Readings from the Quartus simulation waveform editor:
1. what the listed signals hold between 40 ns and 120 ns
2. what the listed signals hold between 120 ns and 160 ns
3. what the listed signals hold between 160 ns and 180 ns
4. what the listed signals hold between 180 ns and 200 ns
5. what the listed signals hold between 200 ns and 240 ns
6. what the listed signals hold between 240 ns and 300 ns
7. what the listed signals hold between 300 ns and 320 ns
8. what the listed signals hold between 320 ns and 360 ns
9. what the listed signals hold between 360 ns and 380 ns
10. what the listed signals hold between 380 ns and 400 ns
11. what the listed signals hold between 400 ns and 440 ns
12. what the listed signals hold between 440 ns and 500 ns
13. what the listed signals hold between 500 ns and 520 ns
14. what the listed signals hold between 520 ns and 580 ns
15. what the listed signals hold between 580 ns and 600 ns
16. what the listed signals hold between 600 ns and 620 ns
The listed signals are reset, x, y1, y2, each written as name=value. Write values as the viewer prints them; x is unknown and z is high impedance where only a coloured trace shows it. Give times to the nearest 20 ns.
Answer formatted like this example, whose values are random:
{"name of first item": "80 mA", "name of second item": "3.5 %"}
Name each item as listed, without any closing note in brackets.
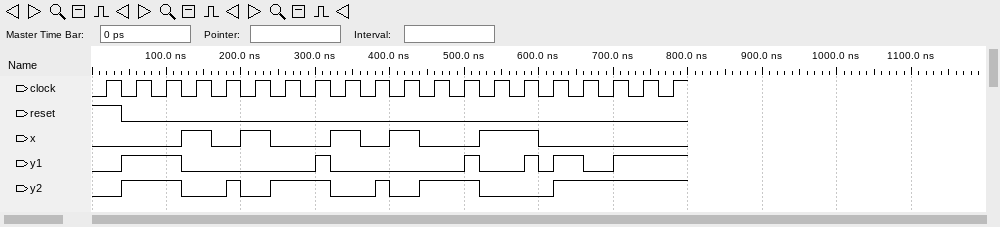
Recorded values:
{"what the listed signals hold between 40 ns and 120 ns": "reset=0, x=0, y1=1, y2=1", "what the listed signals hold between 120 ns and 160 ns": "reset=0, x=1, y1=0, y2=0", "what the listed signals hold between 160 ns and 180 ns": "reset=0, x=0, y1=0, y2=0", "what the listed signals hold between 180 ns and 200 ns": "reset=0, x=0, y1=0, y2=1", "what the listed signals hold between 200 ns and 240 ns": "reset=0, x=1, y1=0, y2=0", "what the listed signals hold between 240 ns and 300 ns": "reset=0, x=0, y1=0, y2=1", "what the listed signals hold between 300 ns and 320 ns": "reset=0, x=0, y1=1, y2=1", "what the listed signals hold between 320 ns and 360 ns": "reset=0, x=1, y1=0, y2=0", "what the listed signals hold between 360 ns and 380 ns": "reset=0, x=0, y1=0, y2=0", "what the listed signals hold between 380 ns and 400 ns": "reset=0, x=0, y1=0, y2=1", "what the listed signals hold between 400 ns and 440 ns": "reset=0, x=1, y1=0, y2=0", "what the listed signals hold between 440 ns and 500 ns": "reset=0, x=0, y1=0, y2=1", "what the listed signals hold between 500 ns and 520 ns": "reset=0, x=0, y1=1, y2=1", "what the listed signals hold between 520 ns and 580 ns": "reset=0, x=1, y1=0, y2=0", "what the listed signals hold between 580 ns and 600 ns": "reset=0, x=1, y1=1, y2=0", "what the listed signals hold between 600 ns and 620 ns": "reset=0, x=0, y1=0, y2=0"}
